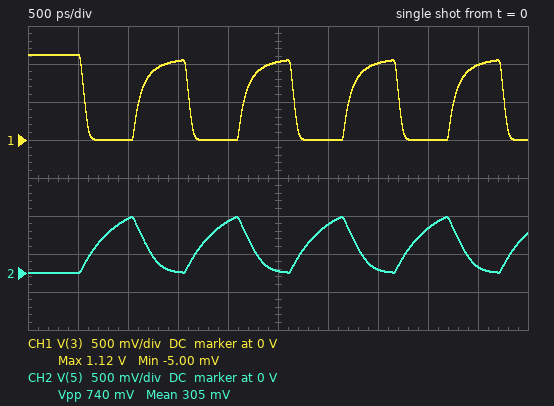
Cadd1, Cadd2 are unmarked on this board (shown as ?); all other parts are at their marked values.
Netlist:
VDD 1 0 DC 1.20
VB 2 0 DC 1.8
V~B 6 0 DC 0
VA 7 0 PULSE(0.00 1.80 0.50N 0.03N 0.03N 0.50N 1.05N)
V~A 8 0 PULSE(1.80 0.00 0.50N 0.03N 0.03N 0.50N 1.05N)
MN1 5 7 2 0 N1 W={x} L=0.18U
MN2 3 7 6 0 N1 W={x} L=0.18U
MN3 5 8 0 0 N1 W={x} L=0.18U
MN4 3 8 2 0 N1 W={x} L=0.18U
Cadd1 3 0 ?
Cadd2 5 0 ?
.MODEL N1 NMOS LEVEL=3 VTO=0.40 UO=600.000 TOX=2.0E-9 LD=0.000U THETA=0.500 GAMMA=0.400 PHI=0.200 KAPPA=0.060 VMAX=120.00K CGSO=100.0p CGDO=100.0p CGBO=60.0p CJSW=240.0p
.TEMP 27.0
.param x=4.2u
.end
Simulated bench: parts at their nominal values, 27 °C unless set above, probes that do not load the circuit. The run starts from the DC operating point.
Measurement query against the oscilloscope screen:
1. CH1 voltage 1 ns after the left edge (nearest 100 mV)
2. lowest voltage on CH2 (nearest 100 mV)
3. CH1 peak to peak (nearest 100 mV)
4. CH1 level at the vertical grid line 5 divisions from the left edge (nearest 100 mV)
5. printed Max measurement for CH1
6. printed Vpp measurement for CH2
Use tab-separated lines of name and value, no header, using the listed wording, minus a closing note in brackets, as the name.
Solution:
CH1 voltage 1 ns after the left edge	0 V
lowest voltage on CH2	0 V
CH1 peak to peak	1.1 V
CH1 level at the vertical grid line 5 divisions from the left edge	1.0 V
printed Max measurement for CH1	1.12 V
printed Vpp measurement for CH2	740 mV
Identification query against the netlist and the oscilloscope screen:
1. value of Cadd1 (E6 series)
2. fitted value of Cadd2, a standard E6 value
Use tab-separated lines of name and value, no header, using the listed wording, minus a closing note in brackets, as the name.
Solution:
value of Cadd1	330 fF
fitted value of Cadd2, a standard E6 value	1.5 pF
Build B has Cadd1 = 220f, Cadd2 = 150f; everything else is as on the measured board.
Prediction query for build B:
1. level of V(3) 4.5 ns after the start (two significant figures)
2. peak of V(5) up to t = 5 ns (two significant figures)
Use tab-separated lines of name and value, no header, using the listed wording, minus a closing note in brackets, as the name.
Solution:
level of V(3) 4.5 ns after the start	1.0 V
peak of V(5) up to t = 5 ns	1.1 V
